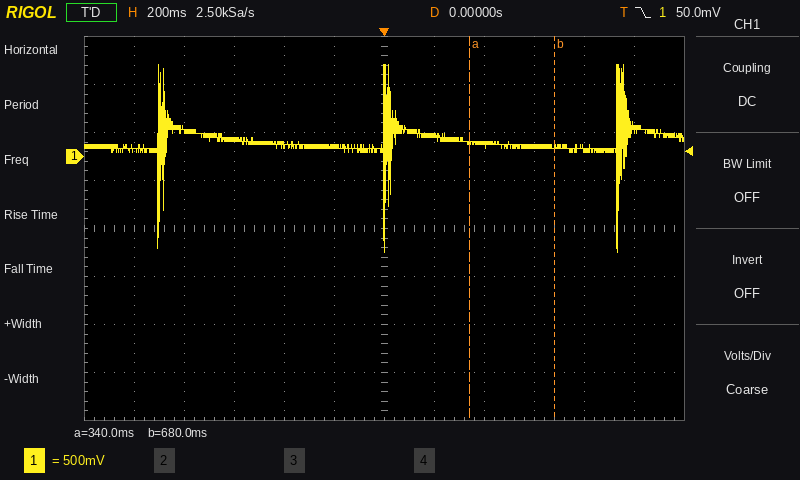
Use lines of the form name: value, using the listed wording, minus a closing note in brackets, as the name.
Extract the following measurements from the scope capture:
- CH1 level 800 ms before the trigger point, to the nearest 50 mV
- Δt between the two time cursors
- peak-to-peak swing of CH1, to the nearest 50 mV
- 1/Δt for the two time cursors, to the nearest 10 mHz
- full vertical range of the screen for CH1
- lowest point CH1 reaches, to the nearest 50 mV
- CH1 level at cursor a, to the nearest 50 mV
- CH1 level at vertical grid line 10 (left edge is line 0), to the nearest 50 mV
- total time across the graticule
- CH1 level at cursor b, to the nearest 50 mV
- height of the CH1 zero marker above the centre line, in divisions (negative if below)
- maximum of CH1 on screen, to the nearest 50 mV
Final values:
CH1 level 800 ms before the trigger point, to the nearest 50 mV: 300 mV
Δt between the two time cursors: 340 ms
peak-to-peak swing of CH1, to the nearest 50 mV: 1.95 V
1/Δt for the two time cursors, to the nearest 10 mHz: 2.94 Hz
full vertical range of the screen for CH1: 4 V
lowest point CH1 reaches, to the nearest 50 mV: -1.00 V
CH1 level at cursor a, to the nearest 50 mV: 150 mV
CH1 level at vertical grid line 10 (left edge is line 0), to the nearest 50 mV: 100 mV
total time across the graticule: 2.4 s
CH1 level at cursor b, to the nearest 50 mV: 100 mV
height of the CH1 zero marker above the centre line, in divisions: +1.5 div
maximum of CH1 on screen, to the nearest 50 mV: 950 mV
